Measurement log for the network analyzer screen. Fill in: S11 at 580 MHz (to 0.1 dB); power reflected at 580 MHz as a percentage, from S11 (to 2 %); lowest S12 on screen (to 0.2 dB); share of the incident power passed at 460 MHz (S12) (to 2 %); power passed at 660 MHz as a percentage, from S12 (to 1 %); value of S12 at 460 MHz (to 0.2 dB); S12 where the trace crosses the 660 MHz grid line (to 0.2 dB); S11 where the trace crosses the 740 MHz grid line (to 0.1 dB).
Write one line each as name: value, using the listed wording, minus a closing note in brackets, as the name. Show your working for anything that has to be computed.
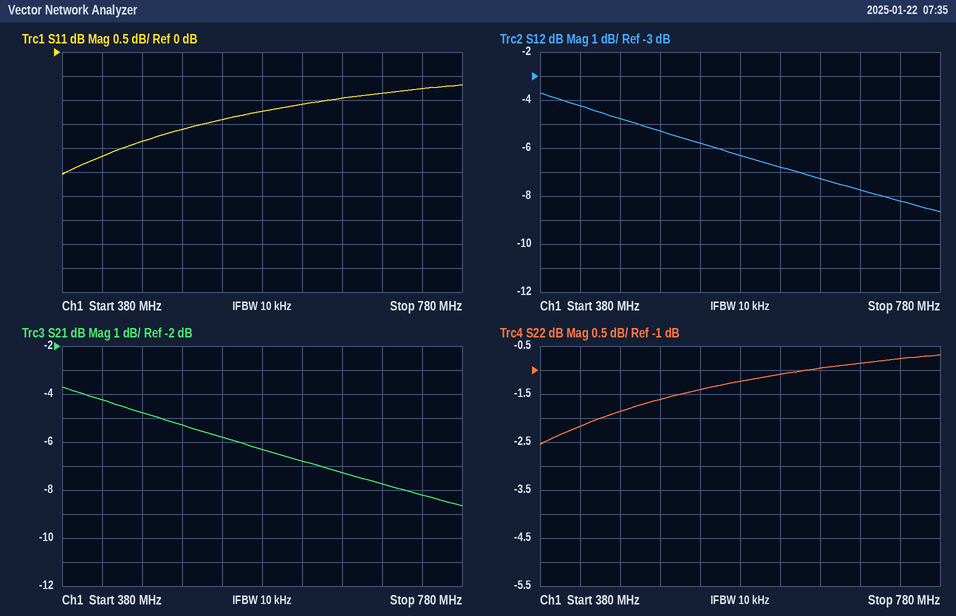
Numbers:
S11 at 580 MHz: -1.2 dB
power reflected at 580 MHz as a percentage, from S11: 10^(-1.2/10) ≈ 76 %
lowest S12 on screen: -8.6 dB
share of the incident power passed at 460 MHz (S12): 10^(-4.8/10) ≈ 33.1 %, so 34 % to the nearest 2 %
power passed at 660 MHz as a percentage, from S12: 10^(-7.2/10) ≈ 19 %
value of S12 at 460 MHz: -4.8 dB
S12 where the trace crosses the 660 MHz grid line: -7.2 dB
S11 where the trace crosses the 740 MHz grid line: -0.8 dB
